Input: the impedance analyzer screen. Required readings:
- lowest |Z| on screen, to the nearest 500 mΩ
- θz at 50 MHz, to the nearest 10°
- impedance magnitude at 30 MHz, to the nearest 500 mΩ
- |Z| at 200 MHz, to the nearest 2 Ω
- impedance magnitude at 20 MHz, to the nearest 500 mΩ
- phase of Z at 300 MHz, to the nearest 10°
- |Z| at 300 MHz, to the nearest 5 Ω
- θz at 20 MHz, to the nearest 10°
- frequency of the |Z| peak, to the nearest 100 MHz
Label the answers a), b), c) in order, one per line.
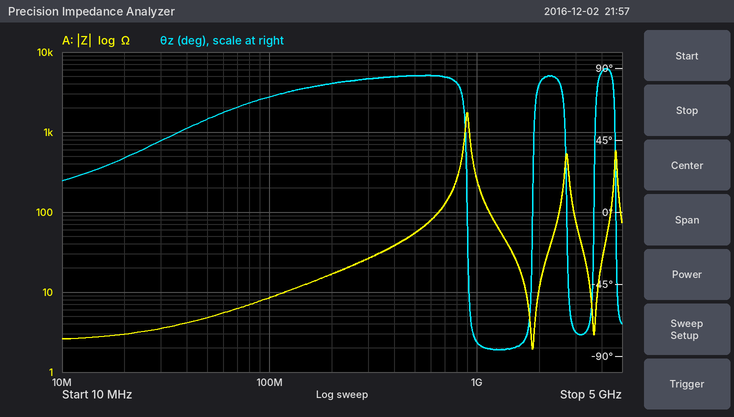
a) 2.0 Ω
b) 60°
c) 3.5 Ω
d) 16 Ω
e) 3.0 Ω
f) 80°
g) 25 Ω
h) 30°
i) 900 MHz
